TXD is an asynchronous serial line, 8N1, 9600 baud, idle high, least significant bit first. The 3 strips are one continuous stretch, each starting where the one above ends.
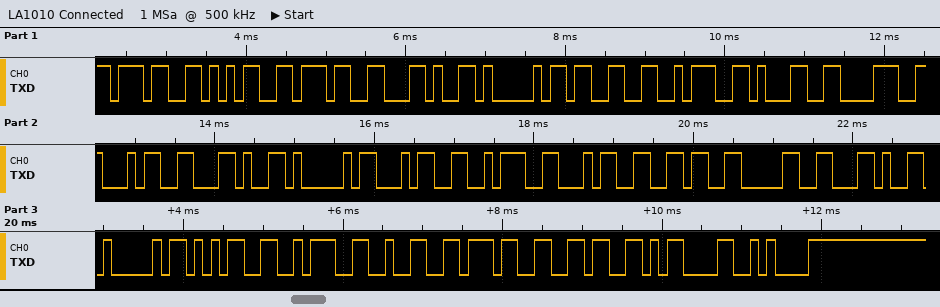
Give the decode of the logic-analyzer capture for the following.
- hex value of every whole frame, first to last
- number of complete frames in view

37 35 37 2C 41 33 3A 31 38 34 2C 41 34 3A 34 36 30 2C 41 35 3A 32 37 36 0D 0A
26
